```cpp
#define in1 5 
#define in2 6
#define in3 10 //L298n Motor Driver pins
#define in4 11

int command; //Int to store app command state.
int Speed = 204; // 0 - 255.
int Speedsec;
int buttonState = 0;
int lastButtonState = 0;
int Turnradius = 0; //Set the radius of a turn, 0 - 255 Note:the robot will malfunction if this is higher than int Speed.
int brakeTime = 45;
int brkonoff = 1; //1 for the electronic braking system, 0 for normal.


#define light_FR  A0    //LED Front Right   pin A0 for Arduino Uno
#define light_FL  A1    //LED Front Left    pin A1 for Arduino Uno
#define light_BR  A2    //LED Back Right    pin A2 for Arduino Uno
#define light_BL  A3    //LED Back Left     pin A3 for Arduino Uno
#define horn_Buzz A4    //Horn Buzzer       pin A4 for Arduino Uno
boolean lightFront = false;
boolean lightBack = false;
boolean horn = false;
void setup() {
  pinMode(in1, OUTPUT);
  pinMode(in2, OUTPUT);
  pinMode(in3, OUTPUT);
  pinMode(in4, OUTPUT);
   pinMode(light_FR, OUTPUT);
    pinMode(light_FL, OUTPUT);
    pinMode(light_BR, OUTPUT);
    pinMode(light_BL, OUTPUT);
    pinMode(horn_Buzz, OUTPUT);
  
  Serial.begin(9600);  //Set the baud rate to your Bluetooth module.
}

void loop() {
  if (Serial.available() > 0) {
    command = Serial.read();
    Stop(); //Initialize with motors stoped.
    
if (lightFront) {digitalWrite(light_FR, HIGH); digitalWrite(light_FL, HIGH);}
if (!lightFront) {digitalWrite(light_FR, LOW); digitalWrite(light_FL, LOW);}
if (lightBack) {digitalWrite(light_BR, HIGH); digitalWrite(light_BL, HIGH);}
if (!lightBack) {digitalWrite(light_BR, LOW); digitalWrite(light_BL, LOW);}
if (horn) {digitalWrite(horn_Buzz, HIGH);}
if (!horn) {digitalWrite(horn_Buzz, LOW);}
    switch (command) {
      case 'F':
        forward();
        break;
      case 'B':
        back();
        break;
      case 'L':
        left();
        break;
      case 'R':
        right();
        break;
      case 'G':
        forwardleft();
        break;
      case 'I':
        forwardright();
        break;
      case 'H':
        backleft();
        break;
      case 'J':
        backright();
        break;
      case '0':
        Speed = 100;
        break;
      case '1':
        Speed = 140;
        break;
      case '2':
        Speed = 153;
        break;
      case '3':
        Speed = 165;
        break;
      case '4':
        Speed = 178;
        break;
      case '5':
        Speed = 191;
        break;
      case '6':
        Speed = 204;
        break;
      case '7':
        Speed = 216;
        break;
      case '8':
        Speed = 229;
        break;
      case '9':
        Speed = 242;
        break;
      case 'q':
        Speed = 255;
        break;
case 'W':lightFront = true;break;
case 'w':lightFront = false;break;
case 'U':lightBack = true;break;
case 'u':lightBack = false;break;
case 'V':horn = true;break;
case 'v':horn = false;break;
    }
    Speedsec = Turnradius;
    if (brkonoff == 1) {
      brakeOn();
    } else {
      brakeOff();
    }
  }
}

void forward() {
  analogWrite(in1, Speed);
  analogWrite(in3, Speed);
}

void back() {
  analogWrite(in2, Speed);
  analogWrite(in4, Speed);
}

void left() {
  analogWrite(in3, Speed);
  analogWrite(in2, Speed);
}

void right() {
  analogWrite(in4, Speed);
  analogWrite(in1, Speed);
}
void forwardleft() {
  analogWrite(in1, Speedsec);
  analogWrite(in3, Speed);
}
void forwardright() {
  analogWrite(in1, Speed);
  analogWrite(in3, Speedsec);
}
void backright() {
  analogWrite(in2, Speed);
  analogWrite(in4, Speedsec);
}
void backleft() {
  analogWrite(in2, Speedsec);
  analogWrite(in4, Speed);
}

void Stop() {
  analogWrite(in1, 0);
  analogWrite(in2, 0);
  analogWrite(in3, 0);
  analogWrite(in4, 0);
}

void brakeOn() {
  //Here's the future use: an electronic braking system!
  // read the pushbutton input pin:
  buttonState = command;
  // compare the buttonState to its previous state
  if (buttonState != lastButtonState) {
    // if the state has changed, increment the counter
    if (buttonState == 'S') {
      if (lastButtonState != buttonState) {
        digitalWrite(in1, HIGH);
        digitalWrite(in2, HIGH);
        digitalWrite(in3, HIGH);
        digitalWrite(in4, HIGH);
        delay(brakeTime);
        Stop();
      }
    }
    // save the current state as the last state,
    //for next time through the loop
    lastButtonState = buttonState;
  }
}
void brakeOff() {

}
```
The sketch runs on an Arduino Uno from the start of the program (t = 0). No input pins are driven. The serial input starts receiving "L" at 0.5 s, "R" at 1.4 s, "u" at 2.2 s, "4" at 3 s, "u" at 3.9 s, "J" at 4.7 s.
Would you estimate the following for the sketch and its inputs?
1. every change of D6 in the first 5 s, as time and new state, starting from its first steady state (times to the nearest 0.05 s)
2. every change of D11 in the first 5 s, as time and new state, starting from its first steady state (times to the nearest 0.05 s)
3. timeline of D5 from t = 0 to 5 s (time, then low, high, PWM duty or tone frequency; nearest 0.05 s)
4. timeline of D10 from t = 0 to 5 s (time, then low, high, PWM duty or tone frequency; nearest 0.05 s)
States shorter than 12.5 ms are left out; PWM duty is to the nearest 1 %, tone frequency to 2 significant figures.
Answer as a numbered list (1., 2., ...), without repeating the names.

1. 0 s low; 0.5 s PWM 80 %; 1.4 s low; 4.7 s PWM 70 %
2. 0 s low; 1.4 s PWM 80 %; 2.2 s low
3. 0 s low; 1.4 s PWM 80 %; 2.2 s low
4. 0 s low; 0.5 s PWM 80 %; 1.4 s low
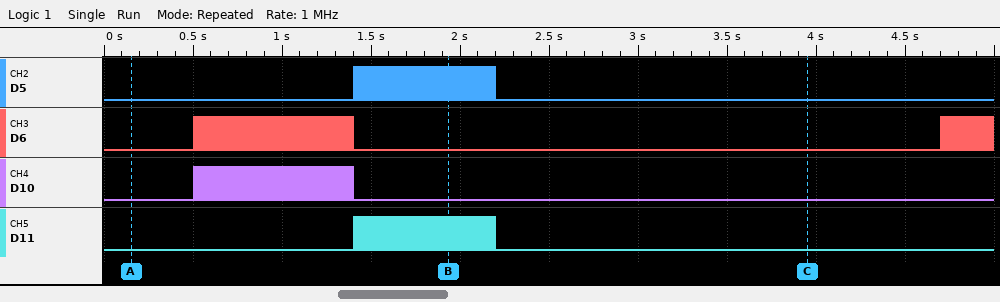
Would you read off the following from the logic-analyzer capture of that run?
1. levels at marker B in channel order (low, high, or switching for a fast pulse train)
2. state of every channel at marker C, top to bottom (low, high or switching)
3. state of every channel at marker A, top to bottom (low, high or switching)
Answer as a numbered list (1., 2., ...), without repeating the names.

1. D5 switching, D6 low, D10 low, D11 switching
2. D5 low, D6 low, D10 low, D11 low
3. D5 low, D6 low, D10 low, D11 low
